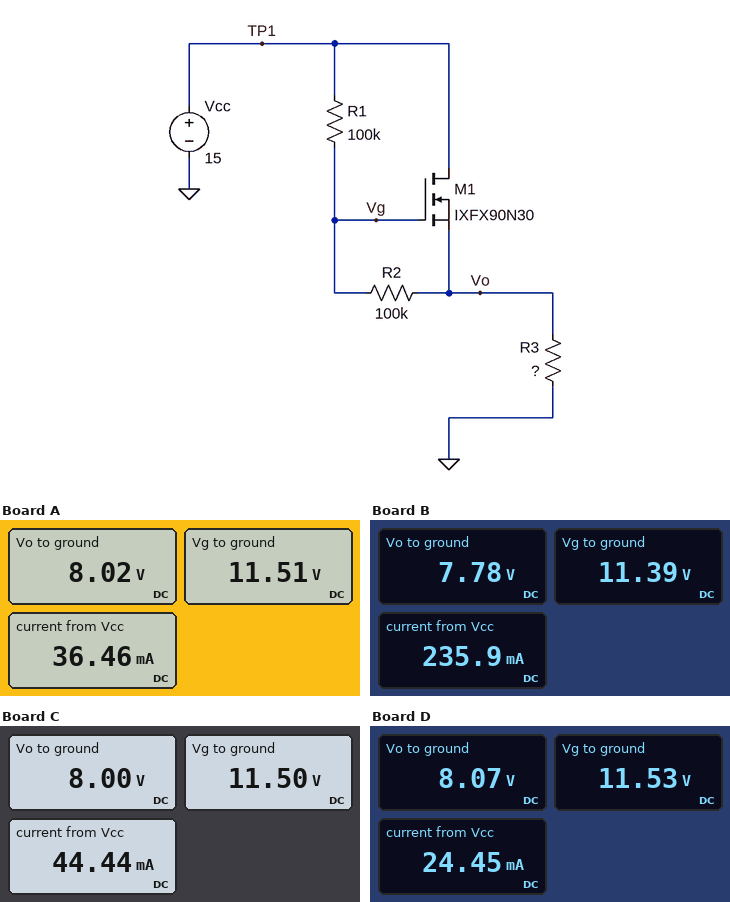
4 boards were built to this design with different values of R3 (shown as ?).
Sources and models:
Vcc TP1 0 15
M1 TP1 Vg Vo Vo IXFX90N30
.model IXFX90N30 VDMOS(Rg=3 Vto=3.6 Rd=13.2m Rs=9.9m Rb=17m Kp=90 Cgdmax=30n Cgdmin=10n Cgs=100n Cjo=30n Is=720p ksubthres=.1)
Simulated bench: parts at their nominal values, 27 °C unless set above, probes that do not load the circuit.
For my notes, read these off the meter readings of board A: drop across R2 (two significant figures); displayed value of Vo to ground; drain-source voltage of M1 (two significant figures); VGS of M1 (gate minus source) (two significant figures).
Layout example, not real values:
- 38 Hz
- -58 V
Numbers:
- 3.5 V
- 8.02 V
- 7.0 V
- 3.5 V
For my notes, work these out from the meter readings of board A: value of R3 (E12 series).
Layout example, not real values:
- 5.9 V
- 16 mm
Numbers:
- 220 Ω
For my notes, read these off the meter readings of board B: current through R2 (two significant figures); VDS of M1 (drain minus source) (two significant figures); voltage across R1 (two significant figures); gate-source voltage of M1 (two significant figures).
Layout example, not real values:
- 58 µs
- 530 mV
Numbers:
- 36 µA
- 7.2 V
- 3.6 V
- 3.6 V
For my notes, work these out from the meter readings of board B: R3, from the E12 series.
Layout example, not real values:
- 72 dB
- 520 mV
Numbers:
- 33 Ω
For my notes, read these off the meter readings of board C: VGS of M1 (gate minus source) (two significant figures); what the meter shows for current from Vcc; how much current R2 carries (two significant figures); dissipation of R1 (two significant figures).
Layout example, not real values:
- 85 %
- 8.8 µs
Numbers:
- 3.5 V
- 44.44 mA
- 35 µA
- 120 µW
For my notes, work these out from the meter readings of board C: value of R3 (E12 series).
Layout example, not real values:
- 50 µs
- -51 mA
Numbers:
- 180 Ω
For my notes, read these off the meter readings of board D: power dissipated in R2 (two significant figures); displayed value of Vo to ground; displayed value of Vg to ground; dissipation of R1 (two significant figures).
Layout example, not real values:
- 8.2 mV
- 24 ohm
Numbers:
- 120 µW
- 8.07 V
- 11.53 V
- 120 µW
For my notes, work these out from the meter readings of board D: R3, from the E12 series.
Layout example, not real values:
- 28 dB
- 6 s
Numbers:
- 330 Ω
